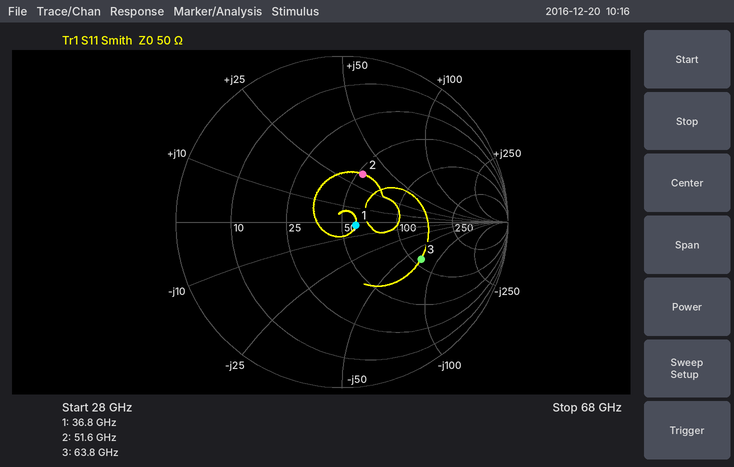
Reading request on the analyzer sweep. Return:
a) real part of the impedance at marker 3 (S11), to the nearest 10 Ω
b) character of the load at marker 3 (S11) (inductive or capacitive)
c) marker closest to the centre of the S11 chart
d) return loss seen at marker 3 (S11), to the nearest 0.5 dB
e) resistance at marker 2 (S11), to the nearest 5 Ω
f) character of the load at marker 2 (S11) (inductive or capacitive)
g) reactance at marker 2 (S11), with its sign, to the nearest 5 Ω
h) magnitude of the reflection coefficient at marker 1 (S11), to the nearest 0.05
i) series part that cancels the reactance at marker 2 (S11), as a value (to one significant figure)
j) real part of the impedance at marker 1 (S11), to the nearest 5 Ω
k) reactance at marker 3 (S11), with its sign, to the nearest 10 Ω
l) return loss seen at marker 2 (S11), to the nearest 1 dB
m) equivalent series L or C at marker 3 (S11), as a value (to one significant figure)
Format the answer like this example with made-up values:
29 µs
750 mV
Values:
110 Ω
capacitive
marker 1
5.5 dB
55 Ω
inductive
+35 Ω
0.10
90 fF
60 Ω
-70 Ω
10 dB
40 fF
